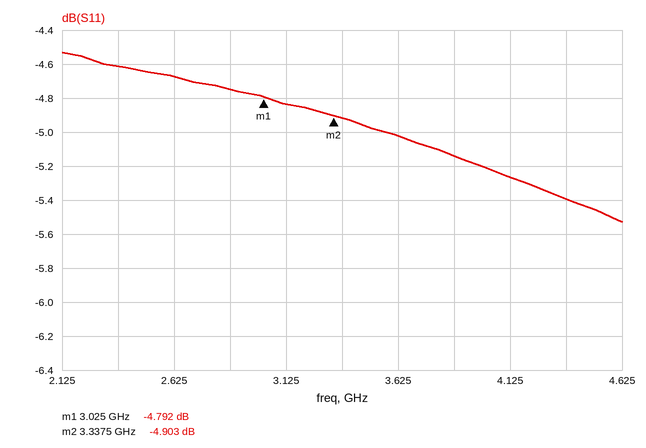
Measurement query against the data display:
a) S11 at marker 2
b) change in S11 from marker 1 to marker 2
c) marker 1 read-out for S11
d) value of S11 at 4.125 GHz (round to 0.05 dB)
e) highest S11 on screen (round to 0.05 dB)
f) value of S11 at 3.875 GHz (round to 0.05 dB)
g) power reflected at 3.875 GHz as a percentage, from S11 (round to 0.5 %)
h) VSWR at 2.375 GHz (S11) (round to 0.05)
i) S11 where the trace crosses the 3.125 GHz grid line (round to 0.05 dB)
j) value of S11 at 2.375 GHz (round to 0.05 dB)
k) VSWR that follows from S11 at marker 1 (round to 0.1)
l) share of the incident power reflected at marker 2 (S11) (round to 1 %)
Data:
-4.903 dB
-0.111 dB
-4.792 dB
-5.25 dB
-4.55 dB
-5.15 dB
30.5 %
3.85
-4.85 dB
-4.60 dB
3.7
32 %
